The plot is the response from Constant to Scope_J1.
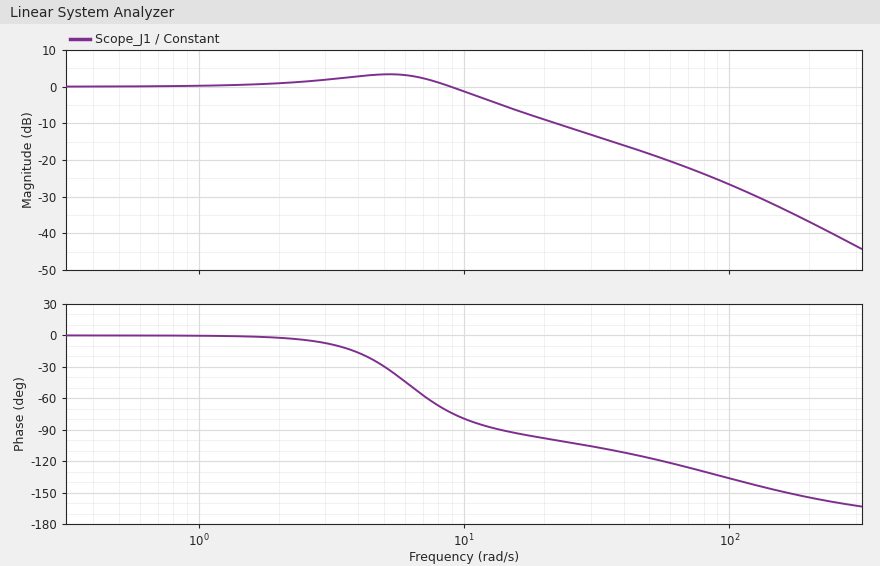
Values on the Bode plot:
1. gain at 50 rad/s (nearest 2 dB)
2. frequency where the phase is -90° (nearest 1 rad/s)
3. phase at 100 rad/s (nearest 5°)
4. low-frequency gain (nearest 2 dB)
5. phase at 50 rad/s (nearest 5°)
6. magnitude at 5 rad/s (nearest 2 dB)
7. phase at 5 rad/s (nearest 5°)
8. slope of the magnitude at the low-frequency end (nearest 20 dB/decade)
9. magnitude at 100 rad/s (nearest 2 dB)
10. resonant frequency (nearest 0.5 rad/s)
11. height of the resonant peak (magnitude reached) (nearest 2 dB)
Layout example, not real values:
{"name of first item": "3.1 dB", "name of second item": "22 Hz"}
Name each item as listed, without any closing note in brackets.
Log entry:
{"gain at 50 rad/s": "-18 dB", "frequency where the phase is -90°": "14 rad/s", "phase at 100 rad/s": "-135°", "low-frequency gain": "0 dB", "phase at 50 rad/s": "-115°", "magnitude at 5 rad/s": "4 dB", "phase at 5 rad/s": "-30°", "slope of the magnitude at the low-frequency end": "0 dB/decade", "magnitude at 100 rad/s": "-26 dB", "resonant frequency": "5.0 rad/s", "height of the resonant peak (magnitude reached)": "4 dB"}
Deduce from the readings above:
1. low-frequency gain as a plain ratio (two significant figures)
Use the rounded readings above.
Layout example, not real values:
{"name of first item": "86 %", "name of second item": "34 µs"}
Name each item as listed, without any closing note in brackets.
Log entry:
{"low-frequency gain as a plain ratio": "1.0"}
